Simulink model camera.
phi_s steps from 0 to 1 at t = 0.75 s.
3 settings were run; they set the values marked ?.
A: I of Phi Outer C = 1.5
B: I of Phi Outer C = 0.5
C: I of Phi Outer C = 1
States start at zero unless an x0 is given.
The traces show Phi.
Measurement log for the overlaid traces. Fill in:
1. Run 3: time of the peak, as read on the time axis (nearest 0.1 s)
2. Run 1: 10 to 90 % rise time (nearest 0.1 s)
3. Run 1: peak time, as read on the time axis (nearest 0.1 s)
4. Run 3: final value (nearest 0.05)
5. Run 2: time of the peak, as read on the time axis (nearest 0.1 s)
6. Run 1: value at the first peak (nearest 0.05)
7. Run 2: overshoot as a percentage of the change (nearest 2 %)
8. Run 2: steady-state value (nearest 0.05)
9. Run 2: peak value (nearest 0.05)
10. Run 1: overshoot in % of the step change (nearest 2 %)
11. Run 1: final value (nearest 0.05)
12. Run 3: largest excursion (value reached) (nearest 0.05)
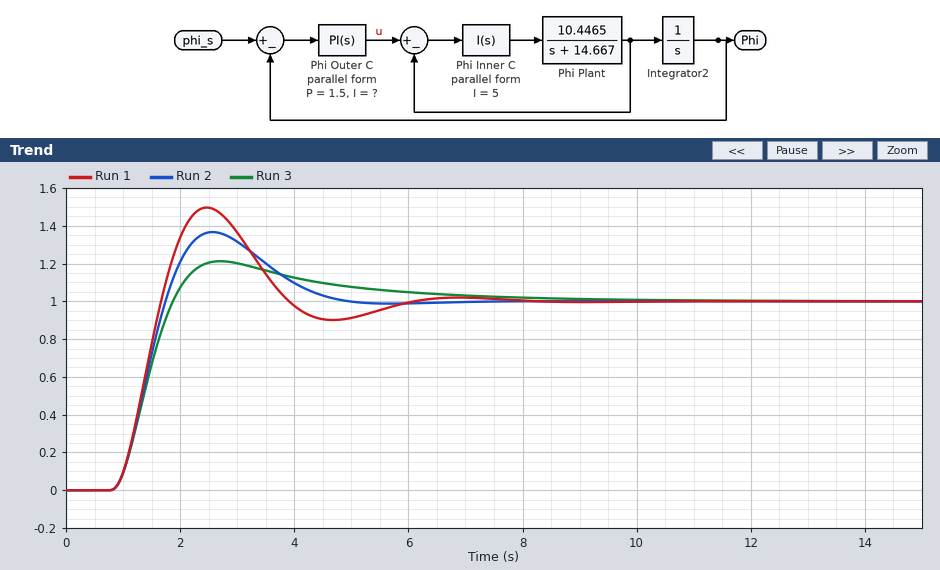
2.7 s
0.6 s
2.5 s
1.00
2.6 s
1.50
36 %
1.00
1.35
50 %
1.00
1.20
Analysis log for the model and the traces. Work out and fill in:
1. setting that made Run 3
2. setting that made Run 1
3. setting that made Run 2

B
A
C
